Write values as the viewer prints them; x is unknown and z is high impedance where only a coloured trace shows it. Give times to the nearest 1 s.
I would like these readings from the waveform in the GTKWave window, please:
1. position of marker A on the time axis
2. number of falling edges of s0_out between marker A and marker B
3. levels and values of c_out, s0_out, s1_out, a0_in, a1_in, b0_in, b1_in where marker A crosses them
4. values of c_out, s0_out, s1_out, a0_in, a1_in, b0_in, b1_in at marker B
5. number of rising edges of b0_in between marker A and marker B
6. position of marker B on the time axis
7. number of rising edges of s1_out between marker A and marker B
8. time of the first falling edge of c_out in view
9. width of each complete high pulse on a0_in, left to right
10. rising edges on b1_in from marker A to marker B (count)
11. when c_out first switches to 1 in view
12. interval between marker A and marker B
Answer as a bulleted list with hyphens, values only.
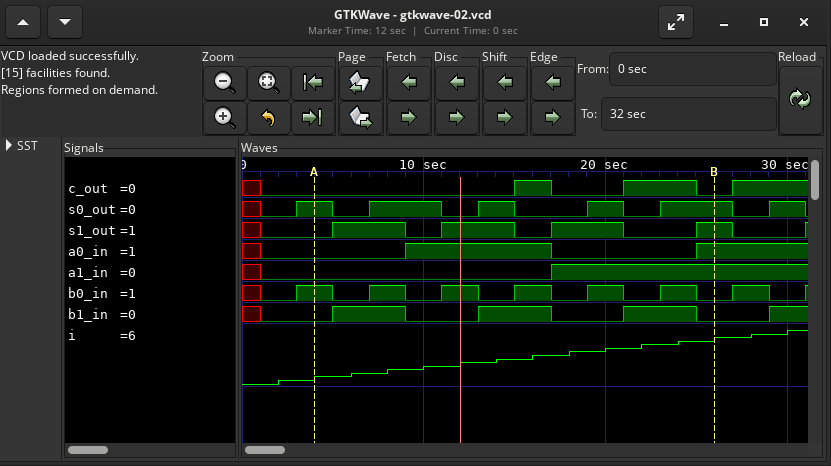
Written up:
- 4 s
- 4
- c_out=0, s0_out=1, s1_out=0, a0_in=0, a1_in=0, b0_in=1, b1_in=0
- c_out=0, s0_out=1, s1_out=1, a0_in=1, a1_in=1, b0_in=0, b1_in=0
- 5
- 26 s
- 4
- 17 s
- 8 s
- 3
- 15 s
- 22 s
